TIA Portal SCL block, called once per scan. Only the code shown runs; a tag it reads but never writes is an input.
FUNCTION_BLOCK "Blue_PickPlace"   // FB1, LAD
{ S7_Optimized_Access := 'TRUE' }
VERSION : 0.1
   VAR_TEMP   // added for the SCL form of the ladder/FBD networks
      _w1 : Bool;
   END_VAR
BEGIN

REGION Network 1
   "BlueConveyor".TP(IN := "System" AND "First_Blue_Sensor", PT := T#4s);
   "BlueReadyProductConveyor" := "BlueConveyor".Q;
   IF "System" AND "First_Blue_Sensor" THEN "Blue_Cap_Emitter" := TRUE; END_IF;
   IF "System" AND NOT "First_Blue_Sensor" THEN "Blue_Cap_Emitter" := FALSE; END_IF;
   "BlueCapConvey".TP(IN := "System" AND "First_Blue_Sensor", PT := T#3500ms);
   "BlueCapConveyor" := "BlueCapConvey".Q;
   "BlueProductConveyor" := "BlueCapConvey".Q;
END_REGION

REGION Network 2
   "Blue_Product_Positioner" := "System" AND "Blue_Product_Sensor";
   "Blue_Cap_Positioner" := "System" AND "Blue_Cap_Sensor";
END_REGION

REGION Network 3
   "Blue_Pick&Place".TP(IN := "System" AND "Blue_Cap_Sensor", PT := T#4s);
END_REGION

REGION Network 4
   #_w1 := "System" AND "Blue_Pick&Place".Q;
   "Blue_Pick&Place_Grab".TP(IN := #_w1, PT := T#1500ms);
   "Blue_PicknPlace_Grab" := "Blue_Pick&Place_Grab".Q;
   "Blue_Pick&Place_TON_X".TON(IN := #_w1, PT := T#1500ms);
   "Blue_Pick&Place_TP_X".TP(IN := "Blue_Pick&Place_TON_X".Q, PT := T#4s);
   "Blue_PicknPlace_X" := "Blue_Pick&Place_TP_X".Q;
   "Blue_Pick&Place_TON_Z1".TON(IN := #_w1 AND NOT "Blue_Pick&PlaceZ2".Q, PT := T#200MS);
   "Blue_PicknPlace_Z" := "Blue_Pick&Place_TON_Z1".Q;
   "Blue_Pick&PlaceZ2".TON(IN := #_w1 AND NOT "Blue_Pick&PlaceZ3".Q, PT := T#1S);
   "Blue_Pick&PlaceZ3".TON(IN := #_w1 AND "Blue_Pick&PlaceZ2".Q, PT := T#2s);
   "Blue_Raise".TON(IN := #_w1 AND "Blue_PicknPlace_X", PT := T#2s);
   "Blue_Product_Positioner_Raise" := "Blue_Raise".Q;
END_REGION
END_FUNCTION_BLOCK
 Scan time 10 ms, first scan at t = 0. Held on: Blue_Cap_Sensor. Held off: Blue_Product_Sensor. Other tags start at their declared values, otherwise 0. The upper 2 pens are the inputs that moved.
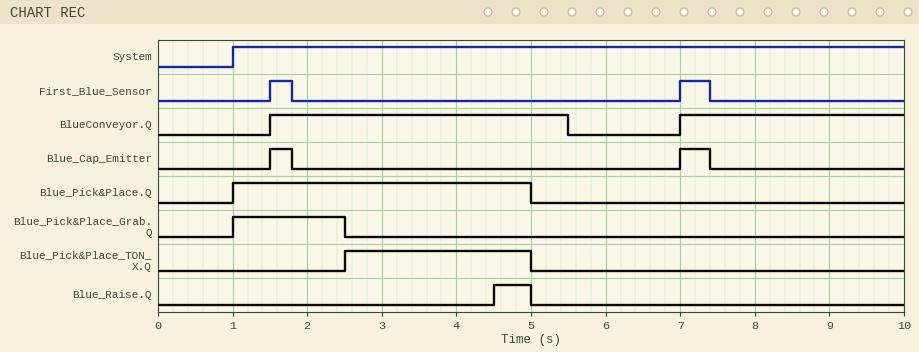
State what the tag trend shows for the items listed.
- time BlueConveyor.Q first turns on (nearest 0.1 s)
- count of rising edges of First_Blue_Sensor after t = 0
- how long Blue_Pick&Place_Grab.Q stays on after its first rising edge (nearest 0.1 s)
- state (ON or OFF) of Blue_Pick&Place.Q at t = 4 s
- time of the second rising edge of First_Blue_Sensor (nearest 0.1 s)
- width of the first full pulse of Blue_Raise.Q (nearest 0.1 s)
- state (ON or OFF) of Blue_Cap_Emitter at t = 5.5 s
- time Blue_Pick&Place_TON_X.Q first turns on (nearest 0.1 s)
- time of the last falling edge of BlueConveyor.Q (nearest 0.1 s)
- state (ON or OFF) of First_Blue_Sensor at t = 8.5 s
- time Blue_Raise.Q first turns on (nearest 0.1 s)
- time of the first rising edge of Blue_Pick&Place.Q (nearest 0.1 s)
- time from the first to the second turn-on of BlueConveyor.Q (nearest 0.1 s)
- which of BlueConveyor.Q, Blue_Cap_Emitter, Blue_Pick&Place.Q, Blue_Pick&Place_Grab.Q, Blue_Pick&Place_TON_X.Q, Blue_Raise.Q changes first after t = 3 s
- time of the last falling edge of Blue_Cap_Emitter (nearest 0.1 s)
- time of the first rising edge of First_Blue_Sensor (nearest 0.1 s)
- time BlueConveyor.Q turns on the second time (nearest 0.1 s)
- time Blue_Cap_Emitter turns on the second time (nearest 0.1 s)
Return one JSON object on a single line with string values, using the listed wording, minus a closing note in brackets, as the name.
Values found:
{"time BlueConveyor.Q first turns on": "1.5 s", "count of rising edges of First_Blue_Sensor after t = 0": "2", "how long Blue_Pick&Place_Grab.Q stays on after its first rising edge": "1.5 s", "state (ON or OFF) of Blue_Pick&Place.Q at t = 4 s": "ON", "time of the second rising edge of First_Blue_Sensor": "7.0 s", "width of the first full pulse of Blue_Raise.Q": "0.5 s", "state (ON or OFF) of Blue_Cap_Emitter at t = 5.5 s": "OFF", "time Blue_Pick&Place_TON_X.Q first turns on": "2.5 s", "time of the last falling edge of BlueConveyor.Q": "5.5 s", "state (ON or OFF) of First_Blue_Sensor at t = 8.5 s": "OFF", "time Blue_Raise.Q first turns on": "4.5 s", "time of the first rising edge of Blue_Pick&Place.Q": "1.0 s", "time from the first to the second turn-on of BlueConveyor.Q": "5.5 s", "which of BlueConveyor.Q, Blue_Cap_Emitter, Blue_Pick&Place.Q, Blue_Pick&Place_Grab.Q, Blue_Pick&Place_TON_X.Q, Blue_Raise.Q changes first after t = 3 s": "Blue_Raise.Q", "time of the last falling edge of Blue_Cap_Emitter": "7.4 s", "time of the first rising edge of First_Blue_Sensor": "1.5 s", "time BlueConveyor.Q turns on the second time": "7.0 s", "time Blue_Cap_Emitter turns on the second time": "7.0 s"}
